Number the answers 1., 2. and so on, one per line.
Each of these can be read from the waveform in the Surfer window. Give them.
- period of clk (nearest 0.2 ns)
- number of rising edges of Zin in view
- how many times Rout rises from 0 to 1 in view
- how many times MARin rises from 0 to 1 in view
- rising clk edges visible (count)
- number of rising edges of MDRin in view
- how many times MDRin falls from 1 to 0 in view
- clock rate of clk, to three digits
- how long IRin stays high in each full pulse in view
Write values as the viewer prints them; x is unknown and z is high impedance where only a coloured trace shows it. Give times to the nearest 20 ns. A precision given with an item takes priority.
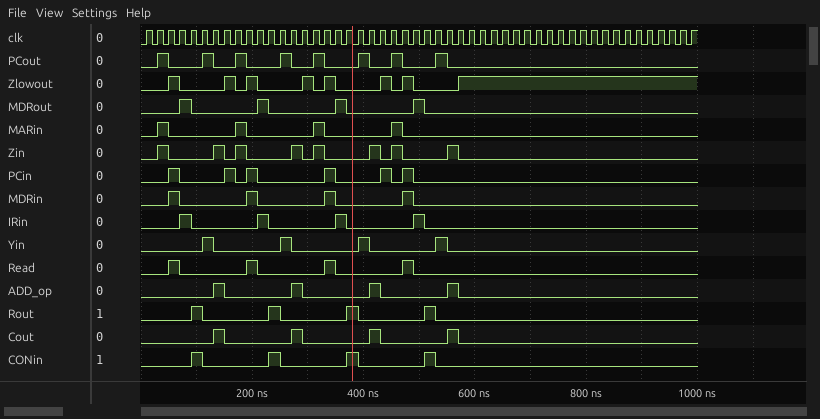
1. 20 ns
2. 8
3. 4
4. 4
5. 50
6. 4
7. 4
8. 50.0 MHz
9. 20 ns, 20 ns, 20 ns, 20 ns
